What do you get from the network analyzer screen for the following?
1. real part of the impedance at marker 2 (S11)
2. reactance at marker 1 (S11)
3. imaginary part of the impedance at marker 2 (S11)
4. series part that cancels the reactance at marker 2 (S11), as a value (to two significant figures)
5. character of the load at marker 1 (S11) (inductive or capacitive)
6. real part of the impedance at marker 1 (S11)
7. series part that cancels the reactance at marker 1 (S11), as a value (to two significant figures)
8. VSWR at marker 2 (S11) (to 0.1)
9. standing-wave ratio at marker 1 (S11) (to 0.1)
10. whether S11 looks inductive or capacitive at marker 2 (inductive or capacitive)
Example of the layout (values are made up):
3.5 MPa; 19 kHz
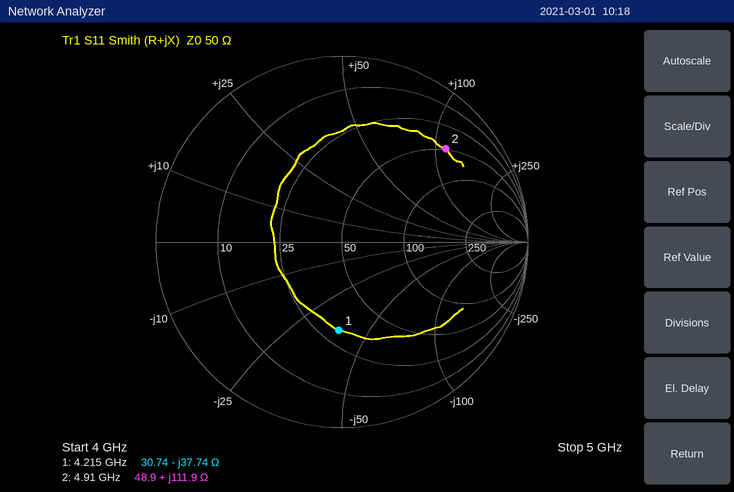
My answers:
48.9 Ω; -37.74 Ω; +111.9 Ω; 290 fF; capacitive; 30.74 Ω; 1.4 nH; 7.0; 2.8; inductive
